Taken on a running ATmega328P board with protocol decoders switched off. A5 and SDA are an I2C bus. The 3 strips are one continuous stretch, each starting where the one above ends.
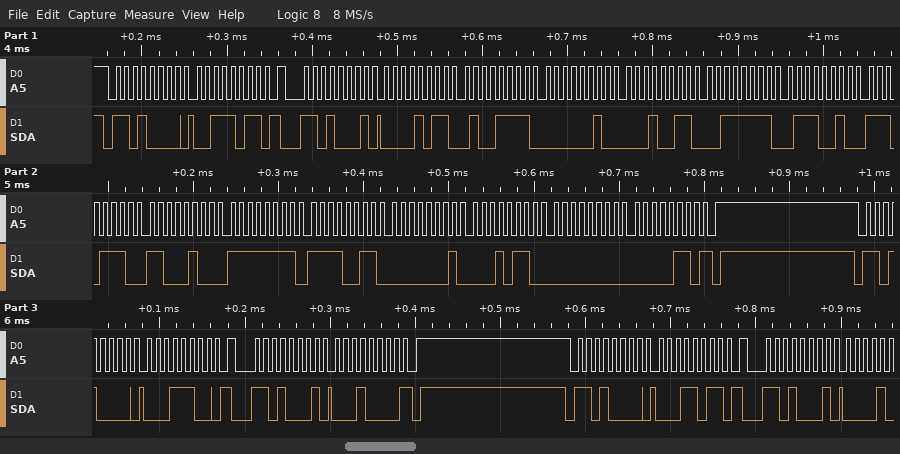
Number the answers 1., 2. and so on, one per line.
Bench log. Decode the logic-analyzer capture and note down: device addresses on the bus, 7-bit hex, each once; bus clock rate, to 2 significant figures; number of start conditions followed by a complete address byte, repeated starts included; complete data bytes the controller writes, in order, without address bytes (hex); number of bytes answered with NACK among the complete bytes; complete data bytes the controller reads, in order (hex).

1. 0x68
2. 100 kHz
3. 6
4. 3B 1C 1B
5. 2
6. 0B 4F 02 13 3F 72 EE C4 FF F3 01 16 00 06 10
